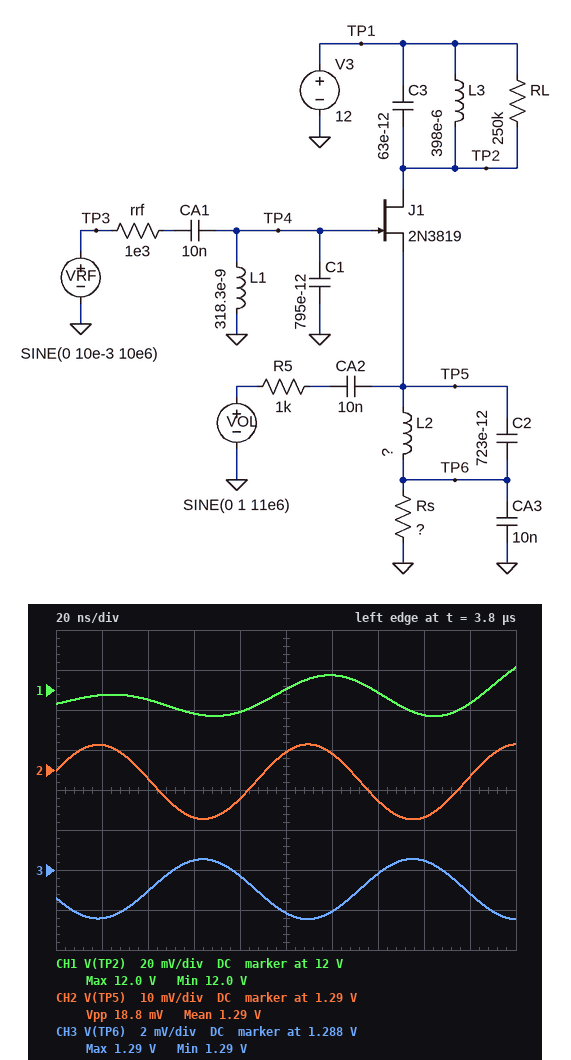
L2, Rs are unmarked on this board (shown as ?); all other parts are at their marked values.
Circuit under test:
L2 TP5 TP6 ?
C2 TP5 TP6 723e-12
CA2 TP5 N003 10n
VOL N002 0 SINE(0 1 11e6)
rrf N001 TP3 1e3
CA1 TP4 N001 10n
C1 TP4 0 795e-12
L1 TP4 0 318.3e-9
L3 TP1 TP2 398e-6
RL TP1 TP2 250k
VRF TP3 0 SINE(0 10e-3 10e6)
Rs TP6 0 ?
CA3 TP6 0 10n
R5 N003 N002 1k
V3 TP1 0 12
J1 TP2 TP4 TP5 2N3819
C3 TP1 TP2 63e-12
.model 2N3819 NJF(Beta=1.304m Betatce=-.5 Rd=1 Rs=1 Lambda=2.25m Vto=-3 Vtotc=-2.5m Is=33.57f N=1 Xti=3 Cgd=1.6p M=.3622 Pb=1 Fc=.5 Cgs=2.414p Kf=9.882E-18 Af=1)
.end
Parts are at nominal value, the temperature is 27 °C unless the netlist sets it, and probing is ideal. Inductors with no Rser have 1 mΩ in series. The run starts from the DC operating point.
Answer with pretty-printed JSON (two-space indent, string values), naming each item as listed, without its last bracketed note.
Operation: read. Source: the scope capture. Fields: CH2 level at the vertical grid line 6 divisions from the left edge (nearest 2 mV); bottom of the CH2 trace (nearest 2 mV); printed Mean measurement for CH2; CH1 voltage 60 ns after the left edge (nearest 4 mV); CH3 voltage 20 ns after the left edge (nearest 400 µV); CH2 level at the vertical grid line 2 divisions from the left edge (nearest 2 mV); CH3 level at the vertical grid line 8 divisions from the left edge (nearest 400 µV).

{
  "CH2 level at the vertical grid line 6 divisions from the left edge": "1.294 V",
  "bottom of the CH2 trace": "1.278 V",
  "printed Mean measurement for CH2": "1.29 V",
  "CH1 voltage 60 ns after the left edge": "11.988 V",
  "CH3 voltage 20 ns after the left edge": "1.2856 V",
  "CH2 level at the vertical grid line 2 divisions from the left edge": "1.288 V",
  "CH3 level at the vertical grid line 8 divisions from the left edge": "1.2884 V"
}
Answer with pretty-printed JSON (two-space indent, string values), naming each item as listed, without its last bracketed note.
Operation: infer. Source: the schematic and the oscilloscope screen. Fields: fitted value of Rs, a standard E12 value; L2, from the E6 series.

{
  "fitted value of Rs, a standard E12 value": "330 Ω",
  "L2, from the E6 series": "100 nH"
}
